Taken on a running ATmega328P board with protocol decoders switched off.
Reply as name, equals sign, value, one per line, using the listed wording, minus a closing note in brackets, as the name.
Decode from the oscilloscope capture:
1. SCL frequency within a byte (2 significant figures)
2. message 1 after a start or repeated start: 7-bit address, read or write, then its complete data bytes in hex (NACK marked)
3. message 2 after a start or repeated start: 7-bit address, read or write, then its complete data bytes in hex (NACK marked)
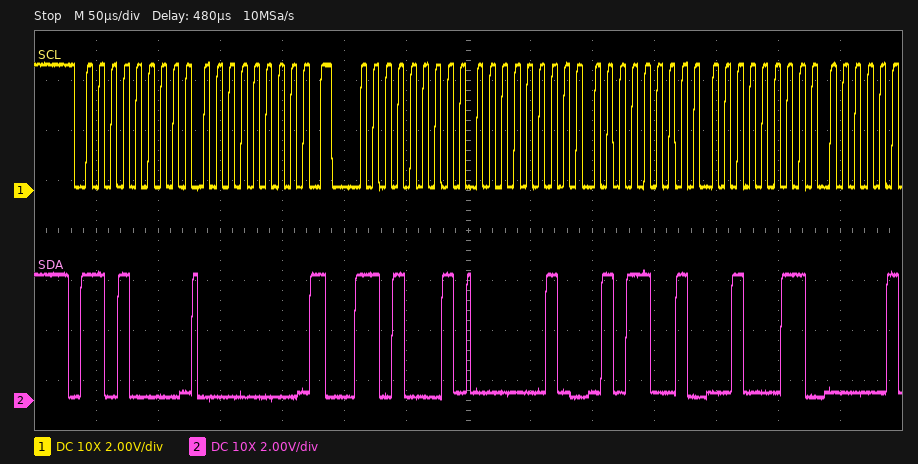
SCL frequency within a byte = 100 kHz
message 1 after a start or repeated start: 7-bit address, read or write, then its complete data bytes in hex = 0x68 write: 00
message 2 after a start or repeated start: 7-bit address, read or write, then its complete data bytes in hex = 0x68 read: 02 59 23
